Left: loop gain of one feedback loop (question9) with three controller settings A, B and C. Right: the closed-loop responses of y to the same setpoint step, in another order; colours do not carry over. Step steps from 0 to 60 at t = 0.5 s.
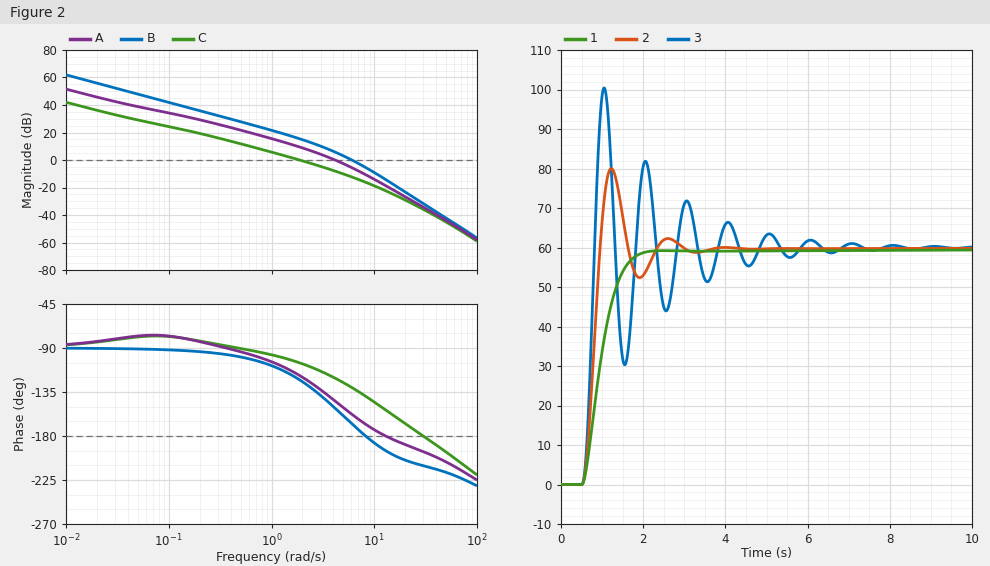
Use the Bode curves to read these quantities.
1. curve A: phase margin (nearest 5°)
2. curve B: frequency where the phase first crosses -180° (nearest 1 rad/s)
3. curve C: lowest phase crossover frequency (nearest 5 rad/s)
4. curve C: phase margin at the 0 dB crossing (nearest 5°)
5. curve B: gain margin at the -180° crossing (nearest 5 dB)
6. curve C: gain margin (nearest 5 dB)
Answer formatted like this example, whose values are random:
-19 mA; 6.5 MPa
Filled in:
35°; 8 rad/s; 30 rad/s; 75°; 5 dB; 35 dB
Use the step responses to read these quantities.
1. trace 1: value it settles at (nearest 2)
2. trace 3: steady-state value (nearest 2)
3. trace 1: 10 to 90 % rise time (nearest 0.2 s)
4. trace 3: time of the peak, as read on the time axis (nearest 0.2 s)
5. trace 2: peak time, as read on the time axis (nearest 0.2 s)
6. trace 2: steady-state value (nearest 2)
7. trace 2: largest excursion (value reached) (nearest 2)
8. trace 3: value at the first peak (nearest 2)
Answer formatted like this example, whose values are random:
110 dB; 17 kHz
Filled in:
60; 60; 0.8 s; 1.0 s; 1.2 s; 60; 80; 100
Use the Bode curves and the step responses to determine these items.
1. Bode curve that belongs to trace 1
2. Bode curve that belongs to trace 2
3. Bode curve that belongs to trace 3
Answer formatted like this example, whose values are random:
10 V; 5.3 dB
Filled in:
C; A; B
